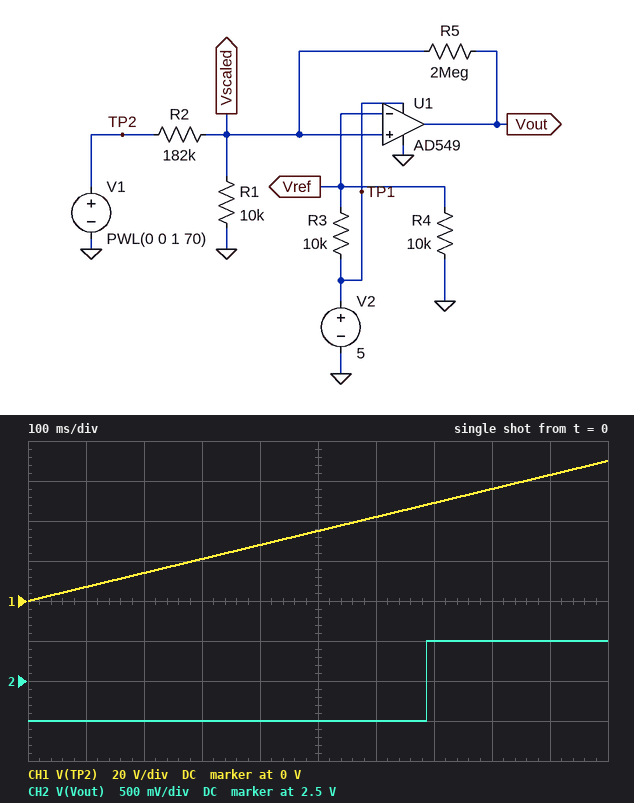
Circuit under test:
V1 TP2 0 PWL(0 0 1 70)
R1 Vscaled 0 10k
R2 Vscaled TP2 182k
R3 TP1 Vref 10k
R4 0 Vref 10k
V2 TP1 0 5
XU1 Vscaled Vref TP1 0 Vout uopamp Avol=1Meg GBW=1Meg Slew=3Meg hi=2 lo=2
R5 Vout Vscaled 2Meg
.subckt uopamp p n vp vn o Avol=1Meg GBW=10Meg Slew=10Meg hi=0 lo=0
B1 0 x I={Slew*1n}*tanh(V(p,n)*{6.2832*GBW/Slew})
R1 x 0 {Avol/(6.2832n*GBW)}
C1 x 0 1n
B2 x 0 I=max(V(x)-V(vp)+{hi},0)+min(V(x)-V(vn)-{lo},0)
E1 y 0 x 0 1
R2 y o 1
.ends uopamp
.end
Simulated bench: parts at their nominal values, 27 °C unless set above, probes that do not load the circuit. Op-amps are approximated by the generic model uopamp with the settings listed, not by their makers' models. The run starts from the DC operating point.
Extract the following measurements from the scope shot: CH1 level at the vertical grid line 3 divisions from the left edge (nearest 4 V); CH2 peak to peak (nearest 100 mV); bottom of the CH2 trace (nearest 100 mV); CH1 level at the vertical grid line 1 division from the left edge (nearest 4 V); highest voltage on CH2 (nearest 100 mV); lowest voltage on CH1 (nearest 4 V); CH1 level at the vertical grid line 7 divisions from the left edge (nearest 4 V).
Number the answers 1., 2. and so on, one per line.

1. 20 V
2. 1.0 V
3. 2.0 V
4. 8 V
5. 3.0 V
6. 0 V
7. 48 V
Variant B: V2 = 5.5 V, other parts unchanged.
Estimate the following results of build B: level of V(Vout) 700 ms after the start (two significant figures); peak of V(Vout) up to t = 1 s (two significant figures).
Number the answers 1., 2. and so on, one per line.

1. 2.0 V
2. 3.5 V
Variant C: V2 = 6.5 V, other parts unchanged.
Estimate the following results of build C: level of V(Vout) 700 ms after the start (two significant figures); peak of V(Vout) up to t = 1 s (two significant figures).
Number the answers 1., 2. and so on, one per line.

1. 2.0 V
2. 4.5 V
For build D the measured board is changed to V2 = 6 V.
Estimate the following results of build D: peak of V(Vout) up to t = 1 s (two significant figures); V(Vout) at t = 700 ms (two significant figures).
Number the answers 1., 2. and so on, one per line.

1. 4.0 V
2. 2.0 V
